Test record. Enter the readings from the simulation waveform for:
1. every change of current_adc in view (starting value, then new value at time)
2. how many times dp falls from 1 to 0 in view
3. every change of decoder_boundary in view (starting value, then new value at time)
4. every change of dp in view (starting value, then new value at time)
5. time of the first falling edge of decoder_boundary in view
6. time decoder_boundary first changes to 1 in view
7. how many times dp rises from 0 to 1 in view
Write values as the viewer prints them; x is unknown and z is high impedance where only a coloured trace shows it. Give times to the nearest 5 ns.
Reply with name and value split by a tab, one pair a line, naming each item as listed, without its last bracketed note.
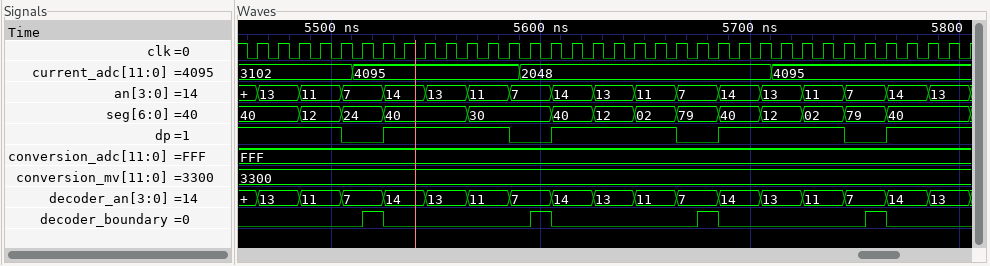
every change of current_adc in view	3102, 4095 at 5510 ns, 2048 at 5590 ns, 4095 at 5710 ns
how many times dp falls from 1 to 0 in view	4
every change of decoder_boundary in view	0, 1 at 5515 ns, 0 at 5525 ns, 1 at 5595 ns, 0 at 5605 ns, 1 at 5675 ns, 0 at 5685 ns, 1 at 5755 ns, 0 at 5765 ns
every change of dp in view	1, 0 at 5505 ns, 1 at 5525 ns, 0 at 5585 ns, 1 at 5605 ns, 0 at 5665 ns, 1 at 5685 ns, 0 at 5745 ns, 1 at 5765 ns
time of the first falling edge of decoder_boundary in view	5525 ns
time decoder_boundary first changes to 1 in view	5515 ns
how many times dp rises from 0 to 1 in view	4
